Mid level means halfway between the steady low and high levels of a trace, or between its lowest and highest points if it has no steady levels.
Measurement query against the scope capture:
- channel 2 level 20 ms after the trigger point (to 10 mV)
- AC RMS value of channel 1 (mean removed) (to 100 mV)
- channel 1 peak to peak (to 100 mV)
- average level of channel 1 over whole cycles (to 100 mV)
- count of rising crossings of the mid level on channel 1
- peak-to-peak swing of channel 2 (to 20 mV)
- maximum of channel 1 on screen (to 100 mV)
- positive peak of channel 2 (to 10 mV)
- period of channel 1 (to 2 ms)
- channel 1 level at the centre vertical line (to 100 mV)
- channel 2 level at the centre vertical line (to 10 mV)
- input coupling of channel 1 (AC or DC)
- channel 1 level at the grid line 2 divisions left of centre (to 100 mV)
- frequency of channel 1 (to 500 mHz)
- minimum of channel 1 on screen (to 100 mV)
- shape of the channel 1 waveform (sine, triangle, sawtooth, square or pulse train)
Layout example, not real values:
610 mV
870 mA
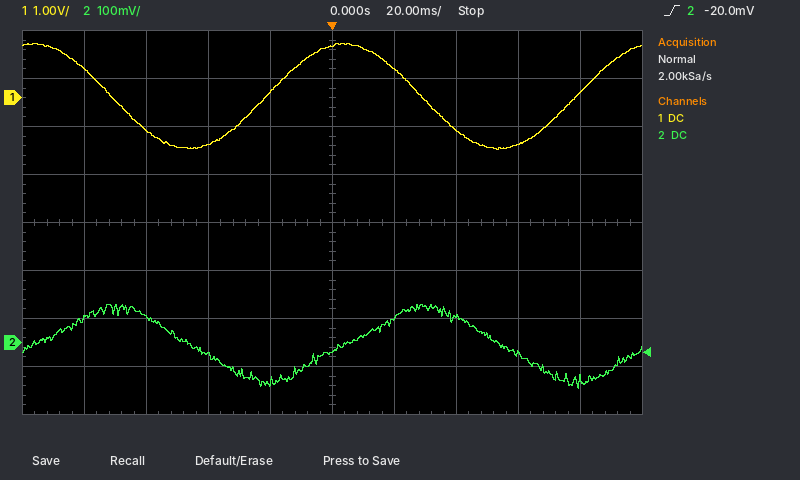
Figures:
50 mV
800 mV
2.2 V
0.0 V
2
180 mV
1.1 V
80 mV
100 ms
1.1 V
-20 mV
DC
-1.0 V
10.0 Hz
-1.1 V
sine
